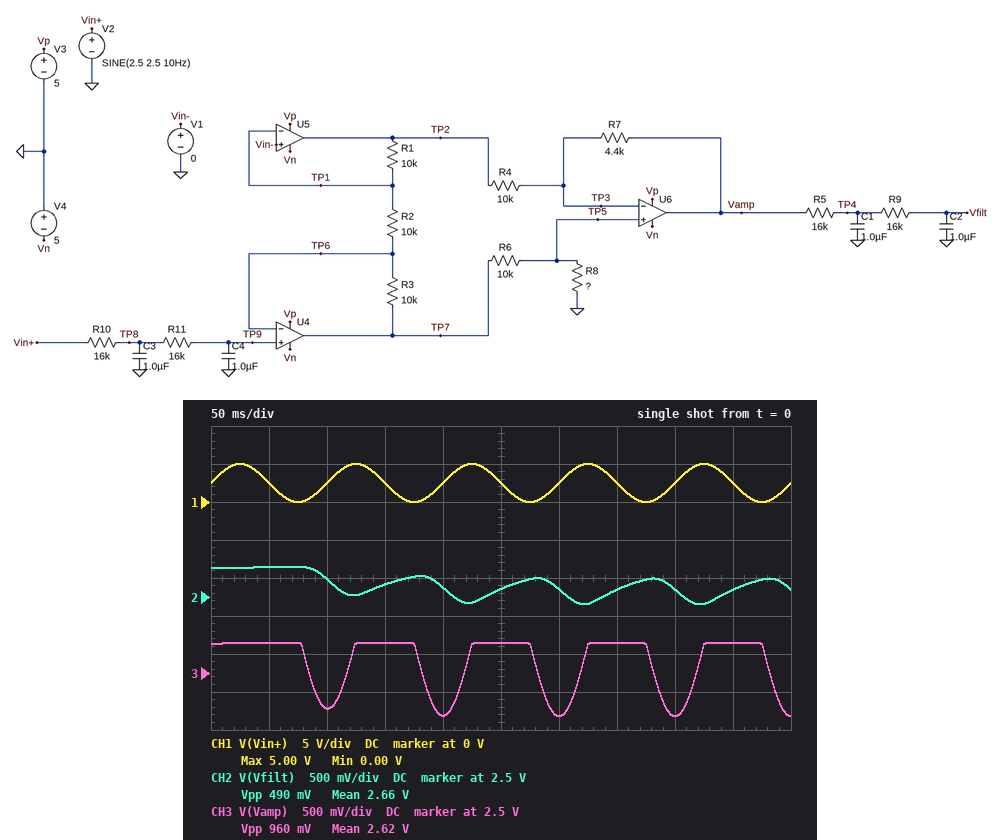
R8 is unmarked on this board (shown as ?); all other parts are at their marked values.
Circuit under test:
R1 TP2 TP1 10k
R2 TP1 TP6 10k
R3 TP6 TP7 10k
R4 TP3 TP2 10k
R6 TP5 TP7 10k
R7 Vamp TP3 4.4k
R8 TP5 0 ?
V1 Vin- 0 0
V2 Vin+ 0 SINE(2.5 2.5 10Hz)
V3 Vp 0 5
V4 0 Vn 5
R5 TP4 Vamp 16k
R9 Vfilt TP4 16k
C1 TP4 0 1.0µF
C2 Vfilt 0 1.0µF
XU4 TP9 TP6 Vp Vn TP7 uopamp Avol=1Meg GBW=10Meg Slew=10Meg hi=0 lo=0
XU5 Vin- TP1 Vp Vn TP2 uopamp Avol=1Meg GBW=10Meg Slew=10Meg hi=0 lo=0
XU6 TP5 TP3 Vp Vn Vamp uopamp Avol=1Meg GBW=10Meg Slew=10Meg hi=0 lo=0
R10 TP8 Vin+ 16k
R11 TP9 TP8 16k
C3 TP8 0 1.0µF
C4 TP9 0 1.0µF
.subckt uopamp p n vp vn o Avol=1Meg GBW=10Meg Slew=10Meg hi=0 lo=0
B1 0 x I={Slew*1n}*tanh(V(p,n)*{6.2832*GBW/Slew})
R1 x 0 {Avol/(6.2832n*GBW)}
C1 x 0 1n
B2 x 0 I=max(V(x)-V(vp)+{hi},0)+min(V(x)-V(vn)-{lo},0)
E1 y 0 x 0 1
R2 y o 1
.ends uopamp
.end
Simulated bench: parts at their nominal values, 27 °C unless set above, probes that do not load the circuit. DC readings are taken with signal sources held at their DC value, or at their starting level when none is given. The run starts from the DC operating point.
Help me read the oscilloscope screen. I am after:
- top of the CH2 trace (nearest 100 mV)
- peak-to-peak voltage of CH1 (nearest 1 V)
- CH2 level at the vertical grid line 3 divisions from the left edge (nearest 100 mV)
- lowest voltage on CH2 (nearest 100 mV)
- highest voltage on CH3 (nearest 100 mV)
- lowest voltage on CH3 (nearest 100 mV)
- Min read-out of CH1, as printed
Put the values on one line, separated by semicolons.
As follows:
2.9 V; 5 V; 2.7 V; 2.4 V; 2.9 V; 1.9 V; 0.00 V
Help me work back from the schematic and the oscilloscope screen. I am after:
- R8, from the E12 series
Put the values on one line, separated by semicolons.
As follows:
3.3 kΩ
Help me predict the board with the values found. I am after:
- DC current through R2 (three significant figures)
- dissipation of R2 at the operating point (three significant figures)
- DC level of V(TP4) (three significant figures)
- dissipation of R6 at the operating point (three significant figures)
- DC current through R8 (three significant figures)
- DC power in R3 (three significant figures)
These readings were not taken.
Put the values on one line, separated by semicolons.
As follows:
250 µA; 625 µW; 2.89 V; 1.41 mW; 376 µA; 625 µW
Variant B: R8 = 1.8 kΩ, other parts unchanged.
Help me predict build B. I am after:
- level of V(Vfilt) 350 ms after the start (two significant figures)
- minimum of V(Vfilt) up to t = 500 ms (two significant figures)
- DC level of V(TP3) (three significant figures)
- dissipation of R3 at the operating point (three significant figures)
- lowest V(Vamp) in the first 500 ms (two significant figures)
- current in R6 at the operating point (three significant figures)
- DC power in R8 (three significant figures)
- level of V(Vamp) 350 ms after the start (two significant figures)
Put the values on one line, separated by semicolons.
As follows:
2.0 V; 1.8 V; 763 mV; 625 µW; 1.5 V; 424 µA; 323 µW; 2.2 V
